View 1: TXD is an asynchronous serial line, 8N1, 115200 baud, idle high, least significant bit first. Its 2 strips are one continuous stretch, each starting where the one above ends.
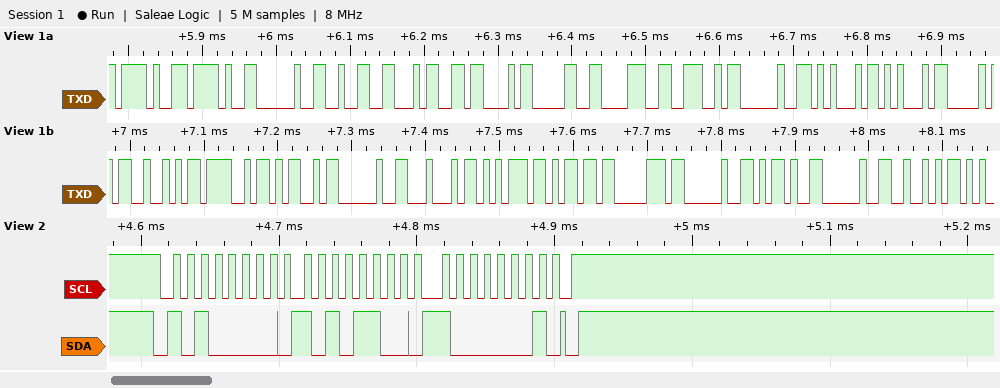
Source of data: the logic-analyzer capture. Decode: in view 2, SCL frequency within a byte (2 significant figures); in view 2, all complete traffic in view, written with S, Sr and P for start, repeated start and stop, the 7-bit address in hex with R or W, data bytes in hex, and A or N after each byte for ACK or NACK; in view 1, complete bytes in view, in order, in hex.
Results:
100 kHz
S 50W A AC A 81 A P
2F 2F 20 32 34 43 30 38 4E 20 45 45 50 52 4F 4D 20 44 75 6D 70 20 2D 20 52
